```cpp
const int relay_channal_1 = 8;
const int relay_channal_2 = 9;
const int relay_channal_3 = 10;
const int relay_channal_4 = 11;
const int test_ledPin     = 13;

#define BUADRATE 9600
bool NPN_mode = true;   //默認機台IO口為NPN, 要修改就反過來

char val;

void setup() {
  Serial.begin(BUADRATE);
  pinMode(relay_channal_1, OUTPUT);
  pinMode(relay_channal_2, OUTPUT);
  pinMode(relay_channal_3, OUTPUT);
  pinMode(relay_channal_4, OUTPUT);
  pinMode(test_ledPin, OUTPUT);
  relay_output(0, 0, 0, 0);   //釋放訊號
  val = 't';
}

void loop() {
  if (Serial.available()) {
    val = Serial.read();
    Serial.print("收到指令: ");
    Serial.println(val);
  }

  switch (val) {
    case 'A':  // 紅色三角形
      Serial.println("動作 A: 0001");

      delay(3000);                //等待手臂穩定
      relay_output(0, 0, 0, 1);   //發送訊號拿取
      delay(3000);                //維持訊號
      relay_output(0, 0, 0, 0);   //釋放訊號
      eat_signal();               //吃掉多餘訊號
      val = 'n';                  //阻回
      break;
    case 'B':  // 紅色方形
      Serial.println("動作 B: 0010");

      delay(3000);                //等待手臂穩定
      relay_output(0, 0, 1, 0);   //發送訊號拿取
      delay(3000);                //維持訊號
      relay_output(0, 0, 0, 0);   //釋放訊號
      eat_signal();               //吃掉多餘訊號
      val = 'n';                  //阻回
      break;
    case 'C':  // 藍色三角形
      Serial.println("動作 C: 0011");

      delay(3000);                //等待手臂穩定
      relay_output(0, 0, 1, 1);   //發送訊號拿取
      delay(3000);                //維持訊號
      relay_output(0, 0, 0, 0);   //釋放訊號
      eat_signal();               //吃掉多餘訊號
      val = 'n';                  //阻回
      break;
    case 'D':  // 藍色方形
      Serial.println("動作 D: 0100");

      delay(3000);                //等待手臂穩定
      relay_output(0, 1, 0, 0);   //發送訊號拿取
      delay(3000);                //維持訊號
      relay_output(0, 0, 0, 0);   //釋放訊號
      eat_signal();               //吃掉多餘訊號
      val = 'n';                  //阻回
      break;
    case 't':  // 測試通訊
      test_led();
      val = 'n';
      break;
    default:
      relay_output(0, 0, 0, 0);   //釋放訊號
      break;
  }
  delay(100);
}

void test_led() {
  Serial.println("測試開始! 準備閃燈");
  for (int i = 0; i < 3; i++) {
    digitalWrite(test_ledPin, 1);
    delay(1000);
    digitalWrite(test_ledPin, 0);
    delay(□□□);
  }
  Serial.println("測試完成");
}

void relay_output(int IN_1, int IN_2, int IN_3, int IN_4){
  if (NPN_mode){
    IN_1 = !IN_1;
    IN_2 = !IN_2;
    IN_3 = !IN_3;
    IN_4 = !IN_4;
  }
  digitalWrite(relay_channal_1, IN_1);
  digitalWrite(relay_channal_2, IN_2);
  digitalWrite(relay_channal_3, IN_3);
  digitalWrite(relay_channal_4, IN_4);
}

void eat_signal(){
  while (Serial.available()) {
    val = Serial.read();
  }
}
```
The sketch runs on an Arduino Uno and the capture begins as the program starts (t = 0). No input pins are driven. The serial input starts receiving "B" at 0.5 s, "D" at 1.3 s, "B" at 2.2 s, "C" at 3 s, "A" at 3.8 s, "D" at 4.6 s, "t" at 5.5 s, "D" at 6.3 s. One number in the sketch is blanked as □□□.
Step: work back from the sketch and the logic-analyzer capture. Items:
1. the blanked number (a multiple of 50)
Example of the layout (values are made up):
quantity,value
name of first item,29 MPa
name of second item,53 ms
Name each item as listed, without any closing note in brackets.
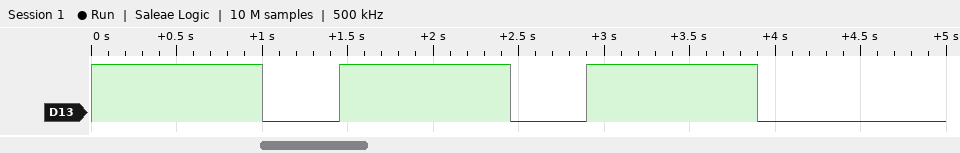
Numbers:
quantity,value
the blanked number,450
